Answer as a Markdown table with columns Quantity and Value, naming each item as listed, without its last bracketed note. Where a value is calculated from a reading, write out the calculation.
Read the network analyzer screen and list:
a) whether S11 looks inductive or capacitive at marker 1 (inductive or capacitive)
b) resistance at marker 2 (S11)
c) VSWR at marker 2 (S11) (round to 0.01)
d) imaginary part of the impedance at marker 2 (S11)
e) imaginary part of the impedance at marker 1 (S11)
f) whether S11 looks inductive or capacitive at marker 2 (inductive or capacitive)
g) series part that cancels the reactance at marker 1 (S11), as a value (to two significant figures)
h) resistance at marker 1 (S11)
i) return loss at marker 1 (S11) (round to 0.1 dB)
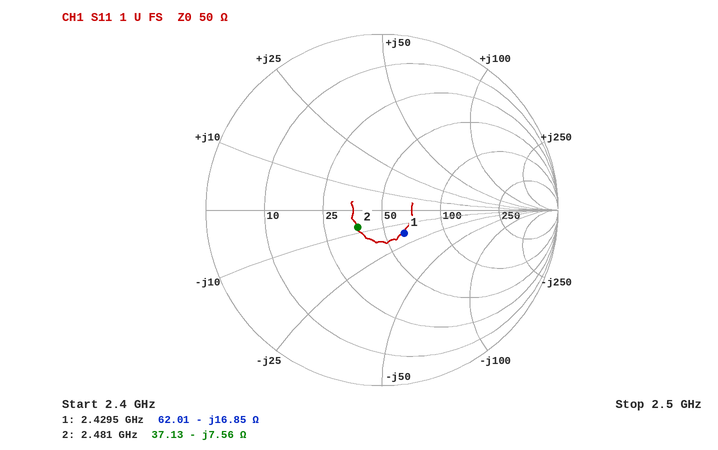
| Quantity | Value |
|---|---|
| whether S11 looks inductive or capacitive at marker 1 | capacitive |
| resistance at marker 2 | 37.13 Ω |
| VSWR at marker 2 (S11) | 1.41 |
| imaginary part of the impedance at marker 2 | -7.56 Ω |
| imaginary part of the impedance at marker 1 | -16.85 Ω |
| whether S11 looks inductive or capacitive at marker 2 | capacitive |
| series part that cancels the reactance at marker 1 (S11), as a value | L = 16.85 Ω/(2π × 2.4295 GHz) ≈ 1.1 nH |
| resistance at marker 1 | 62.01 Ω |
| return loss at marker 1 (S11) | 14.8 dB |
